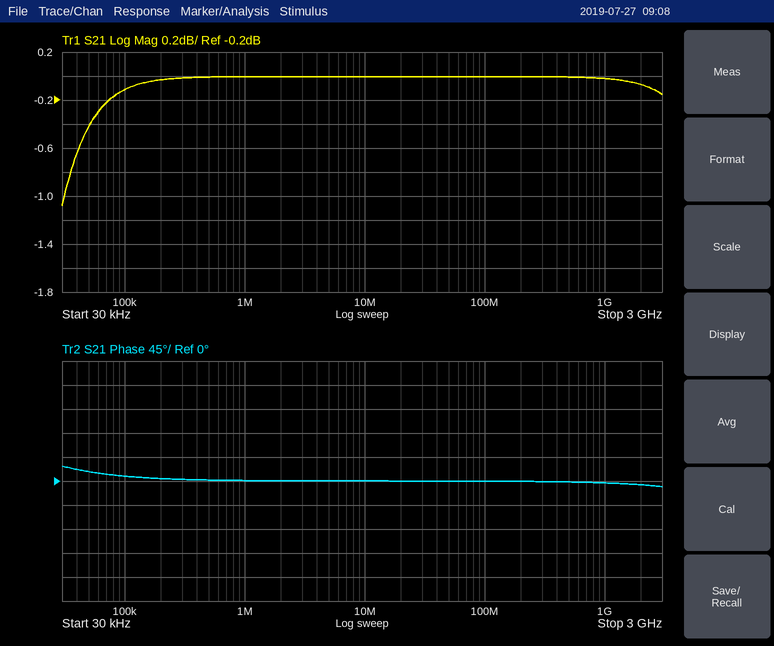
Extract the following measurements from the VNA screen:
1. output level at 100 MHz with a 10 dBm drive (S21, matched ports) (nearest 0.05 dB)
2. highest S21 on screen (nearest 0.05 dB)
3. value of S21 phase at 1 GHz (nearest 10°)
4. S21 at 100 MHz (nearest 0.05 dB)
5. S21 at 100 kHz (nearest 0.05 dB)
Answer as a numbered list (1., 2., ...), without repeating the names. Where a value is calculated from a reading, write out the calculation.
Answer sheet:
1. 10 dBm + (0.00 dB) = 10.00 dBm
2. 0.00 dB
3. 0°
4. 0.00 dB
5. -0.10 dB
